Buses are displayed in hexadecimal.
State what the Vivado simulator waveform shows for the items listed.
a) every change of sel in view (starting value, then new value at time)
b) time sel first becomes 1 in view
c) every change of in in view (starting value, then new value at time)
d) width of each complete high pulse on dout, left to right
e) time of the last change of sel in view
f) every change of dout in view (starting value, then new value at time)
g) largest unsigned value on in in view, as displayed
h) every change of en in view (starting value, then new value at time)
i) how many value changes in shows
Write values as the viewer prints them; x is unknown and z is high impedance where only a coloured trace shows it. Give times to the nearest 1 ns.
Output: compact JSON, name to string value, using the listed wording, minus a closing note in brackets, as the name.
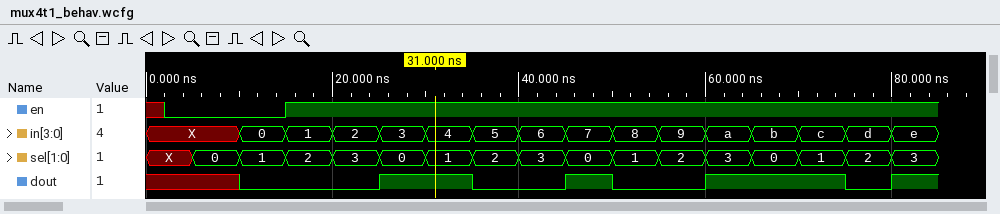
{"every change of sel in view": "X, 0 at 5 ns, 1 at 10 ns, 2 at 15 ns, 3 at 20 ns, 0 at 25 ns, 1 at 30 ns, 2 at 35 ns, 3 at 40 ns, 0 at 45 ns, 1 at 50 ns, 2 at 55 ns, 3 at 60 ns, 0 at 65 ns, 1 at 70 ns, 2 at 75 ns, 3 at 80 ns", "time sel first becomes 1 in view": "10 ns", "every change of in in view": "X, 0 at 10 ns, 1 at 15 ns, 2 at 20 ns, 3 at 25 ns, 4 at 30 ns, 5 at 35 ns, 6 at 40 ns, 7 at 45 ns, 8 at 50 ns, 9 at 55 ns, a at 60 ns, b at 65 ns, c at 70 ns, d at 75 ns, e at 80 ns", "width of each complete high pulse on dout, left to right": "10 ns, 5 ns, 15 ns", "time of the last change of sel in view": "80 ns", "every change of dout in view": "x, 0 at 10 ns, 1 at 25 ns, 0 at 35 ns, 1 at 45 ns, 0 at 50 ns, 1 at 60 ns, 0 at 75 ns, 1 at 80 ns", "largest unsigned value on in in view, as displayed": "e", "every change of en in view": "x, 0 at 2 ns, 1 at 15 ns", "how many value changes in shows": "15"}
